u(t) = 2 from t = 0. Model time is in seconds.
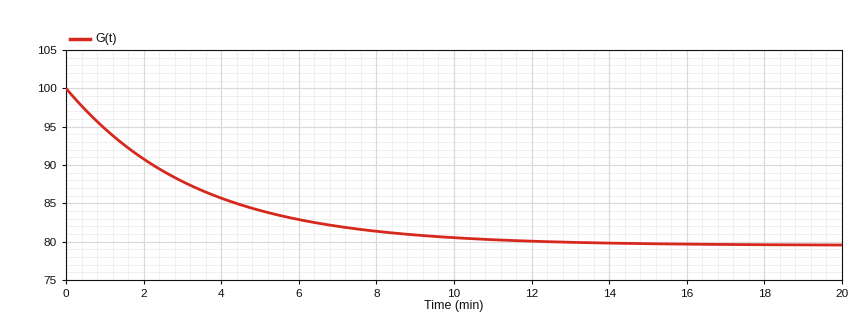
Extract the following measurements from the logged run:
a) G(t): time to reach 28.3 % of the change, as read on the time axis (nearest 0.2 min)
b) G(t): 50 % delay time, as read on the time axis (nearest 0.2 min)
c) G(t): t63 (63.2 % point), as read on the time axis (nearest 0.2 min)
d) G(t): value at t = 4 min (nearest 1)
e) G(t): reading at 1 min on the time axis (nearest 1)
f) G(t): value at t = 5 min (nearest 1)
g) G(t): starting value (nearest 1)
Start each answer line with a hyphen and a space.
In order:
- 1.2 min
- 2.4 min
- 3.4 min
- 86
- 95
- 84
- 100
